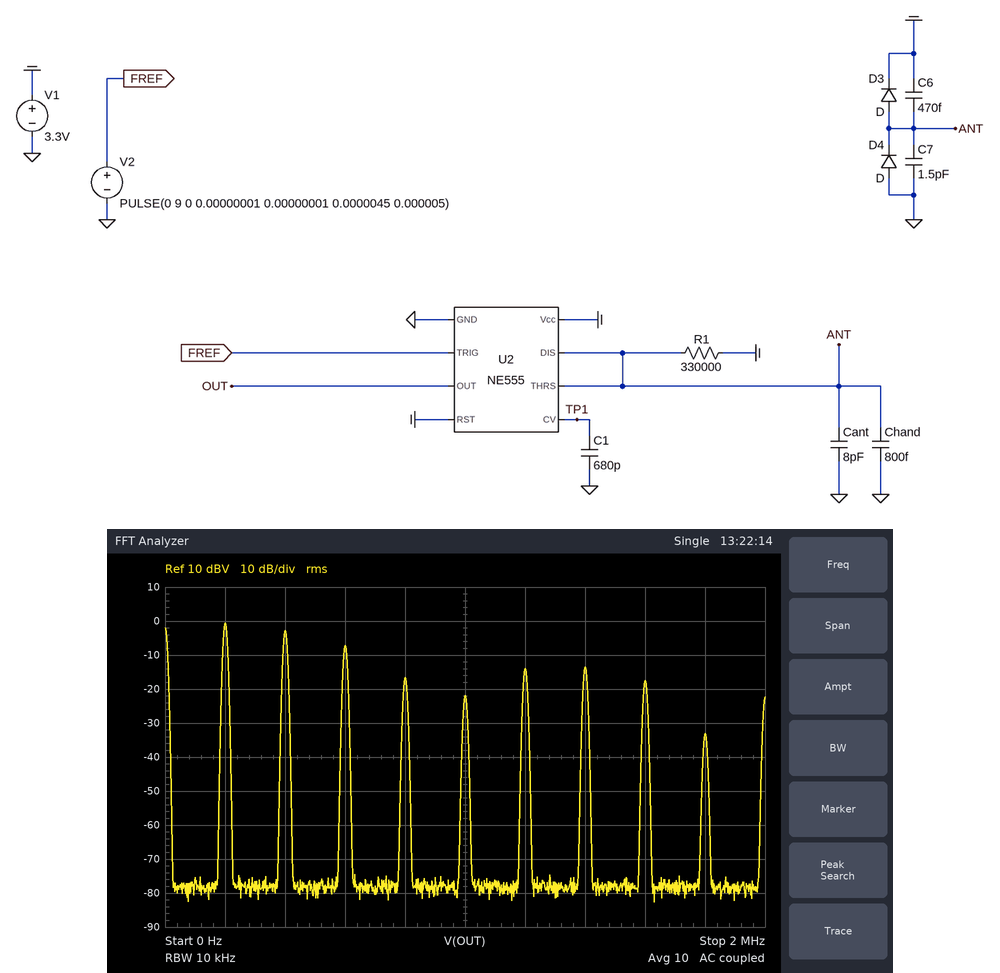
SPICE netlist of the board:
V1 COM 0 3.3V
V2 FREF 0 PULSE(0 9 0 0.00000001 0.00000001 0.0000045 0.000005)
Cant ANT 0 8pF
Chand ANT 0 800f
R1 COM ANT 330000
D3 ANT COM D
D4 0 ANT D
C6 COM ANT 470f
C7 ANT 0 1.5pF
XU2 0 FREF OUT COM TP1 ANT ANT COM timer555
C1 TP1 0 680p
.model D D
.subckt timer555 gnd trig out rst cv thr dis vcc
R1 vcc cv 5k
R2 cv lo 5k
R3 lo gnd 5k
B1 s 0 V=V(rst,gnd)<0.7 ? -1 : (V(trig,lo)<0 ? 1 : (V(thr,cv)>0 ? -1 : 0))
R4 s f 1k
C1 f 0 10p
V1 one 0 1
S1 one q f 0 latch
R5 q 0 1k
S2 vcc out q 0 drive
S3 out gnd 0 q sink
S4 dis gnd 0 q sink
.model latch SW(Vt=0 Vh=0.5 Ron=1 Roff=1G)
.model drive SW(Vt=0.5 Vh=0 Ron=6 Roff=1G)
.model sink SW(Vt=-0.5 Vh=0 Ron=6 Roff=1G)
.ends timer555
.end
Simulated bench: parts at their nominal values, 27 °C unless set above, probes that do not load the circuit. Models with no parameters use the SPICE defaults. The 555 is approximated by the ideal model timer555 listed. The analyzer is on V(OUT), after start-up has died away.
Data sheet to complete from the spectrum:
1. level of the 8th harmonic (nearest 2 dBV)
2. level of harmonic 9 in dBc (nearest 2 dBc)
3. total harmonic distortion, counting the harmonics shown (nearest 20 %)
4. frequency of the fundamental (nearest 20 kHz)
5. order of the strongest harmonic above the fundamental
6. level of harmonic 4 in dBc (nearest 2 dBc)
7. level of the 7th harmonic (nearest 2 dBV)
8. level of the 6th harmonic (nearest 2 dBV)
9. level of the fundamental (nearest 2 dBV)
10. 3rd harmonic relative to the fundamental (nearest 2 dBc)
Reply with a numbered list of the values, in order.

1. -18 dBV
2. -32 dBc
3. 100 %
4. 200 kHz
5. 2
6. -16 dBc
7. -14 dBV
8. -14 dBV
9. 0 dBV
10. -6 dBc
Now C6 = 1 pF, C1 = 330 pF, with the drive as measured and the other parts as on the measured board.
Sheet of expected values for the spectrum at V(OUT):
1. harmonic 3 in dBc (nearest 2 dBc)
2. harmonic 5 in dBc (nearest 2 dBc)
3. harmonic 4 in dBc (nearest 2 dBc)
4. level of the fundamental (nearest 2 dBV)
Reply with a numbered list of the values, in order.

1. -4 dBc
2. -18 dBc
3. -8 dBc
4. -2 dBV
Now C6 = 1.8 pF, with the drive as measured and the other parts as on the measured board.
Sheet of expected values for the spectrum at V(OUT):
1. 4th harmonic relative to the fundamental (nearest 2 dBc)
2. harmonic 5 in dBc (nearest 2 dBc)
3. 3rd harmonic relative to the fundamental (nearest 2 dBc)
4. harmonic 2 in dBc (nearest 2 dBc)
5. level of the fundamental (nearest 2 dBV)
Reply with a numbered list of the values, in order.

1. -4 dBc
2. -6 dBc
3. -2 dBc
4. 0 dBc
5. -6 dBV
